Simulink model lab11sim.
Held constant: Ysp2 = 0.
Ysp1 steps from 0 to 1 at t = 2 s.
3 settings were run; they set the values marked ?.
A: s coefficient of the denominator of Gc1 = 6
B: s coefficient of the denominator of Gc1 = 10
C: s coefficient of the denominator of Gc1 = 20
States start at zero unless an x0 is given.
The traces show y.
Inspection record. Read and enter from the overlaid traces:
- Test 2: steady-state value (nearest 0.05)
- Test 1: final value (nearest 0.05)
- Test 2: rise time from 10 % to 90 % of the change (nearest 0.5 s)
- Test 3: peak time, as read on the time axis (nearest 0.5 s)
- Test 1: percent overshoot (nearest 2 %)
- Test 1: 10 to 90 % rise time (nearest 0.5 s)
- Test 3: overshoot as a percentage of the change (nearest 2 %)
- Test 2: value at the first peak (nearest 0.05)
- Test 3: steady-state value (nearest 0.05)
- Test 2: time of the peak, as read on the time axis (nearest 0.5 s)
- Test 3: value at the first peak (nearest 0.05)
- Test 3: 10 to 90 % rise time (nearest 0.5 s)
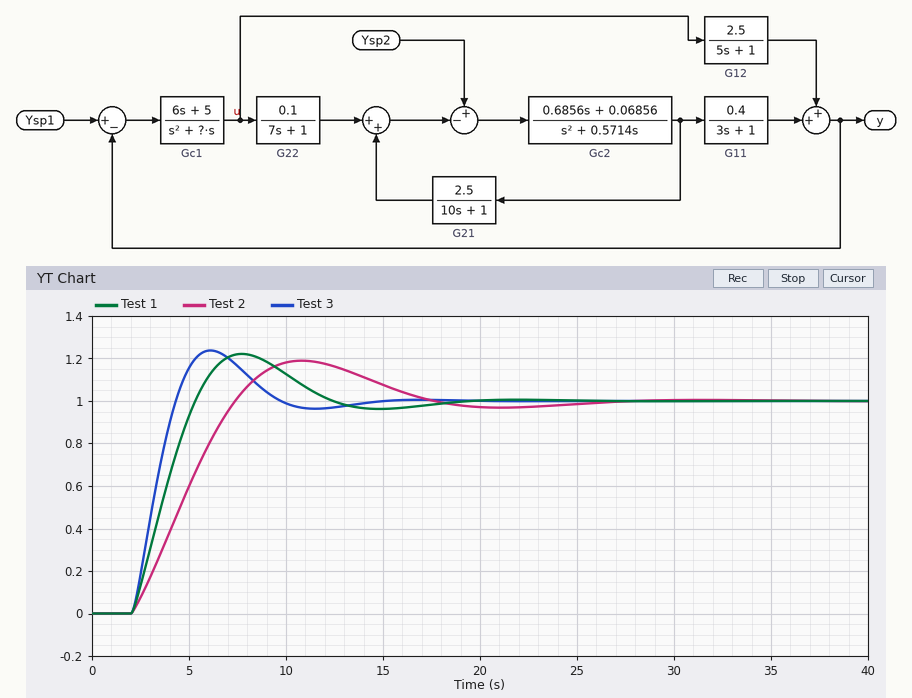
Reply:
1.00
1.00
4.0 s
6.0 s
22 %
2.5 s
24 %
1.20
1.00
11.0 s
1.25
1.5 s
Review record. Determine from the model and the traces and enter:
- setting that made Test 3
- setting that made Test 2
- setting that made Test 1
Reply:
A
C
B
